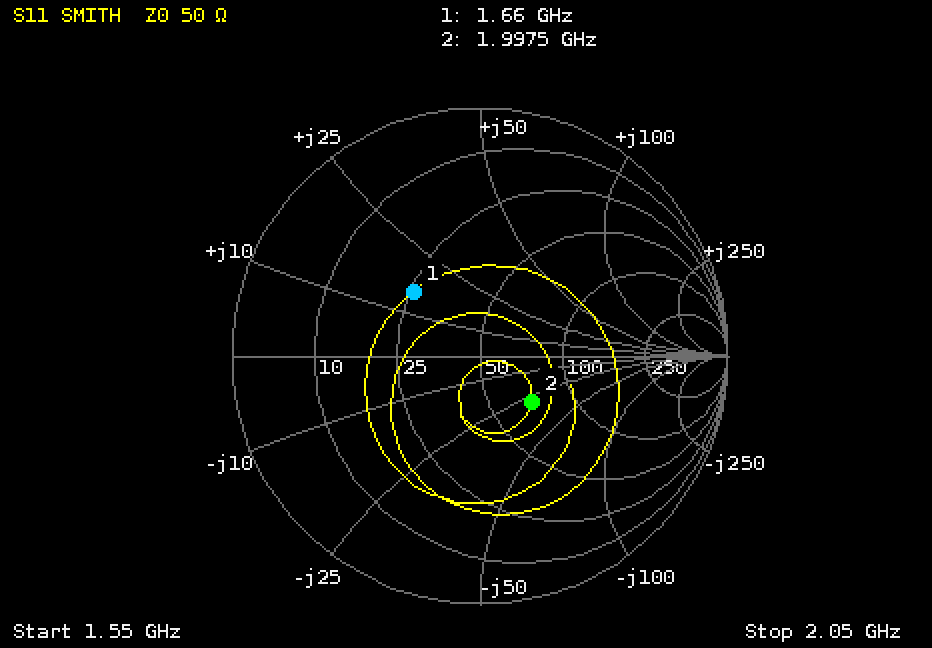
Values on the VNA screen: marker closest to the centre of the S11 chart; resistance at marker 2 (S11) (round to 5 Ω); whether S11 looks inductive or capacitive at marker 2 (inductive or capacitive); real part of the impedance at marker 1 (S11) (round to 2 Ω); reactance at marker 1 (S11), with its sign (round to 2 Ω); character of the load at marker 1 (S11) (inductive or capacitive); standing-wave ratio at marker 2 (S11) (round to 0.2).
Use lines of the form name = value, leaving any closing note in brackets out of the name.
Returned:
marker closest to the centre of the S11 chart = marker 2
resistance at marker 2 (S11) = 70 Ω
whether S11 looks inductive or capacitive at marker 2 = capacitive
real part of the impedance at marker 1 (S11) = 26 Ω
reactance at marker 1 (S11), with its sign = +16 Ω
character of the load at marker 1 (S11) = inductive
standing-wave ratio at marker 2 (S11) = 1.8
